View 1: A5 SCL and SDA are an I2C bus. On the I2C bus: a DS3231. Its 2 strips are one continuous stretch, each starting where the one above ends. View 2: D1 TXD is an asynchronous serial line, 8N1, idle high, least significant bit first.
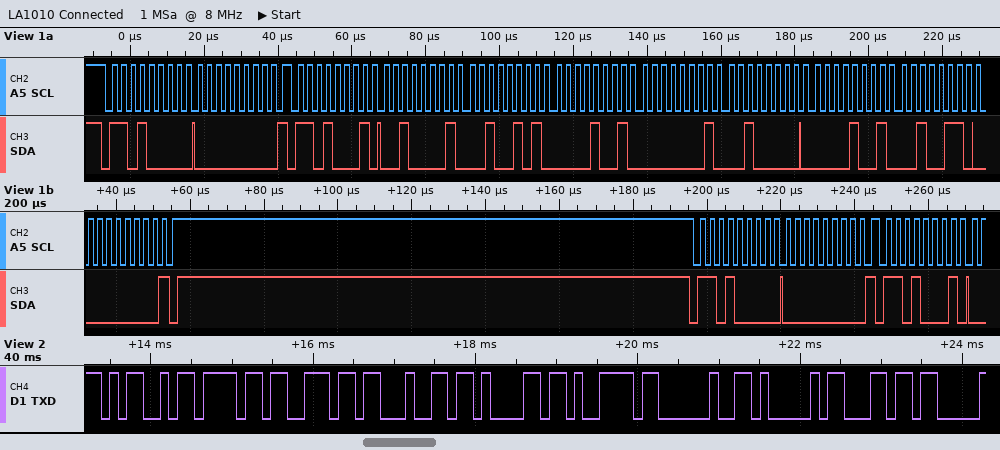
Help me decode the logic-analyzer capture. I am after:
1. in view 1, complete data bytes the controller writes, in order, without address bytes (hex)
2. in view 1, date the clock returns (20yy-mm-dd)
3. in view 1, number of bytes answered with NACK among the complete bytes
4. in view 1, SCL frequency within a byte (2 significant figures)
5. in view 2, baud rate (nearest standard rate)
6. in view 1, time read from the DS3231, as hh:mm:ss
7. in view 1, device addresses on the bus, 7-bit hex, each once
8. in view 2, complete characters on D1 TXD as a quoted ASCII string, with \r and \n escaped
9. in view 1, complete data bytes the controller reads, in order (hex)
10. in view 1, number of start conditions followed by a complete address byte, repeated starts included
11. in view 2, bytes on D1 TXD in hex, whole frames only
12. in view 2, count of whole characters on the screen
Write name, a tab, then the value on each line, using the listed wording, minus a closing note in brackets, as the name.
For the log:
in view 1, complete data bytes the controller writes, in order, without address bytes	00 00
in view 1, date the clock returns	2026-09-20
in view 1, number of bytes answered with NACK among the complete bytes	1
in view 1, SCL frequency within a byte	400 kHz
in view 2, baud rate	9600 baud
in view 1, time read from the DS3231, as hh:mm:ss	09:25:21
in view 1, device addresses on the bus, 7-bit hex, each once	0x68
in view 2, complete characters on D1 TXD as a quoted ASCII string, with \r and \n escaped	"Monday Al"
in view 1, complete data bytes the controller reads, in order	21 25 09 01 20 09 26 00
in view 1, number of start conditions followed by a complete address byte, repeated starts included	4
in view 2, bytes on D1 TXD in hex, whole frames only	0x4D 0x6F 0x6E 0x64 0x61 0x79 0x20 0x41 0x6C
in view 2, count of whole characters on the screen	9
